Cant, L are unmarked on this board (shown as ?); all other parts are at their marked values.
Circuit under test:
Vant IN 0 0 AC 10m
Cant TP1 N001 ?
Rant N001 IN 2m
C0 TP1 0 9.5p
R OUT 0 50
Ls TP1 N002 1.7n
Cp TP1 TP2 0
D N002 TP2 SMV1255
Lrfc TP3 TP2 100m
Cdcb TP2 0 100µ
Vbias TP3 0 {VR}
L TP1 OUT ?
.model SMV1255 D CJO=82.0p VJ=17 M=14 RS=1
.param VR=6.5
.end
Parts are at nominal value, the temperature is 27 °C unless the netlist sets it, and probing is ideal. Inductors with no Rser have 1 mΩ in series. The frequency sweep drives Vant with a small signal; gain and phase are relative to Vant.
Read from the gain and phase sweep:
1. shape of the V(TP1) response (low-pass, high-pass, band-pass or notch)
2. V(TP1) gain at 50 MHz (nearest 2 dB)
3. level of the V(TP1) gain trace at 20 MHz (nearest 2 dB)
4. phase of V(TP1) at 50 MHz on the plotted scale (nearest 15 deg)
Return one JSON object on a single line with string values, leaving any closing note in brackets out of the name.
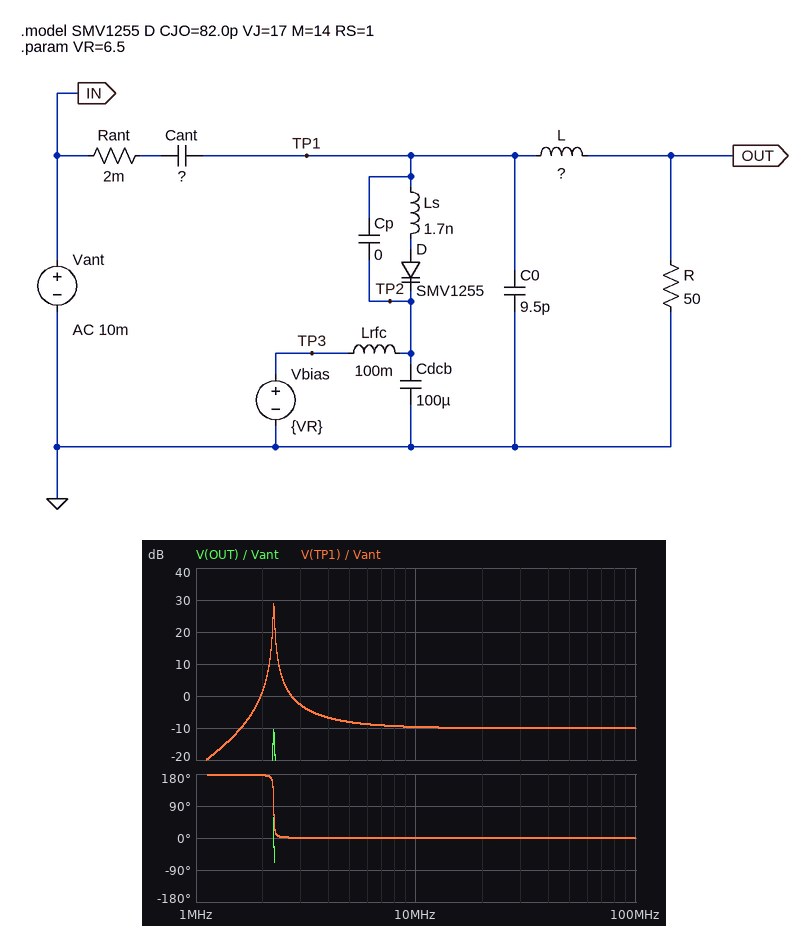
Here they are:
{"shape of the V(TP1) response": "band-pass", "V(TP1) gain at 50 MHz": "-10 dB", "level of the V(TP1) gain trace at 20 MHz": "-10 dB", "phase of V(TP1) at 50 MHz on the plotted scale": "0 deg"}
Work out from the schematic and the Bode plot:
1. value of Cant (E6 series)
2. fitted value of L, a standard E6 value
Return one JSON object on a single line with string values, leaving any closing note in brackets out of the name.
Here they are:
{"value of Cant": "4.7 pF", "fitted value of L, a standard E6 value": "330 µH"}
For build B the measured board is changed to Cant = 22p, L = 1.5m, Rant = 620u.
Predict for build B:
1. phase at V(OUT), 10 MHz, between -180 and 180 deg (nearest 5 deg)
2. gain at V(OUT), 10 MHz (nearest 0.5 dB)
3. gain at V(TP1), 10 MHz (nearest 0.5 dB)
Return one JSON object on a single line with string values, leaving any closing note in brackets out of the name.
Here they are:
{"phase at V(OUT), 10 MHz, between -180 and 180 deg": "-90 deg", "gain at V(OUT), 10 MHz": "-69.0 dB", "gain at V(TP1), 10 MHz": "-3.5 dB"}
